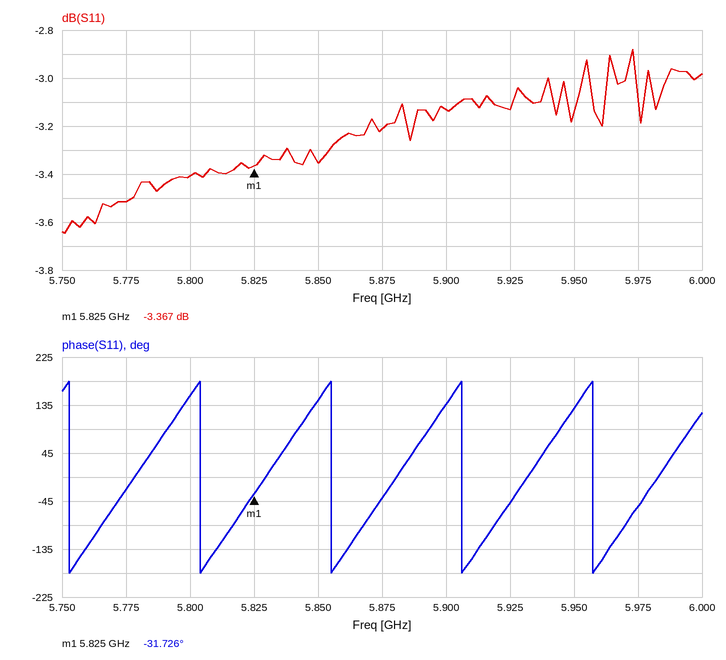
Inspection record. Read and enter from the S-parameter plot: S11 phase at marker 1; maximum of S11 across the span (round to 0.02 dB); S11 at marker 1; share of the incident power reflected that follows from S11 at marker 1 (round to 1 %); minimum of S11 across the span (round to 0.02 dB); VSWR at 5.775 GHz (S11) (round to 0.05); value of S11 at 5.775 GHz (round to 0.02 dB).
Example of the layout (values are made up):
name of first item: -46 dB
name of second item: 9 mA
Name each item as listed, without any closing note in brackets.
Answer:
S11 phase at marker 1: -31.726°
maximum of S11 across the span: -2.88 dB
S11 at marker 1: -3.367 dB
share of the incident power reflected that follows from S11 at marker 1: 46 %
minimum of S11 across the span: -3.64 dB
VSWR at 5.775 GHz (S11): 5.00
value of S11 at 5.775 GHz: -3.52 dB
